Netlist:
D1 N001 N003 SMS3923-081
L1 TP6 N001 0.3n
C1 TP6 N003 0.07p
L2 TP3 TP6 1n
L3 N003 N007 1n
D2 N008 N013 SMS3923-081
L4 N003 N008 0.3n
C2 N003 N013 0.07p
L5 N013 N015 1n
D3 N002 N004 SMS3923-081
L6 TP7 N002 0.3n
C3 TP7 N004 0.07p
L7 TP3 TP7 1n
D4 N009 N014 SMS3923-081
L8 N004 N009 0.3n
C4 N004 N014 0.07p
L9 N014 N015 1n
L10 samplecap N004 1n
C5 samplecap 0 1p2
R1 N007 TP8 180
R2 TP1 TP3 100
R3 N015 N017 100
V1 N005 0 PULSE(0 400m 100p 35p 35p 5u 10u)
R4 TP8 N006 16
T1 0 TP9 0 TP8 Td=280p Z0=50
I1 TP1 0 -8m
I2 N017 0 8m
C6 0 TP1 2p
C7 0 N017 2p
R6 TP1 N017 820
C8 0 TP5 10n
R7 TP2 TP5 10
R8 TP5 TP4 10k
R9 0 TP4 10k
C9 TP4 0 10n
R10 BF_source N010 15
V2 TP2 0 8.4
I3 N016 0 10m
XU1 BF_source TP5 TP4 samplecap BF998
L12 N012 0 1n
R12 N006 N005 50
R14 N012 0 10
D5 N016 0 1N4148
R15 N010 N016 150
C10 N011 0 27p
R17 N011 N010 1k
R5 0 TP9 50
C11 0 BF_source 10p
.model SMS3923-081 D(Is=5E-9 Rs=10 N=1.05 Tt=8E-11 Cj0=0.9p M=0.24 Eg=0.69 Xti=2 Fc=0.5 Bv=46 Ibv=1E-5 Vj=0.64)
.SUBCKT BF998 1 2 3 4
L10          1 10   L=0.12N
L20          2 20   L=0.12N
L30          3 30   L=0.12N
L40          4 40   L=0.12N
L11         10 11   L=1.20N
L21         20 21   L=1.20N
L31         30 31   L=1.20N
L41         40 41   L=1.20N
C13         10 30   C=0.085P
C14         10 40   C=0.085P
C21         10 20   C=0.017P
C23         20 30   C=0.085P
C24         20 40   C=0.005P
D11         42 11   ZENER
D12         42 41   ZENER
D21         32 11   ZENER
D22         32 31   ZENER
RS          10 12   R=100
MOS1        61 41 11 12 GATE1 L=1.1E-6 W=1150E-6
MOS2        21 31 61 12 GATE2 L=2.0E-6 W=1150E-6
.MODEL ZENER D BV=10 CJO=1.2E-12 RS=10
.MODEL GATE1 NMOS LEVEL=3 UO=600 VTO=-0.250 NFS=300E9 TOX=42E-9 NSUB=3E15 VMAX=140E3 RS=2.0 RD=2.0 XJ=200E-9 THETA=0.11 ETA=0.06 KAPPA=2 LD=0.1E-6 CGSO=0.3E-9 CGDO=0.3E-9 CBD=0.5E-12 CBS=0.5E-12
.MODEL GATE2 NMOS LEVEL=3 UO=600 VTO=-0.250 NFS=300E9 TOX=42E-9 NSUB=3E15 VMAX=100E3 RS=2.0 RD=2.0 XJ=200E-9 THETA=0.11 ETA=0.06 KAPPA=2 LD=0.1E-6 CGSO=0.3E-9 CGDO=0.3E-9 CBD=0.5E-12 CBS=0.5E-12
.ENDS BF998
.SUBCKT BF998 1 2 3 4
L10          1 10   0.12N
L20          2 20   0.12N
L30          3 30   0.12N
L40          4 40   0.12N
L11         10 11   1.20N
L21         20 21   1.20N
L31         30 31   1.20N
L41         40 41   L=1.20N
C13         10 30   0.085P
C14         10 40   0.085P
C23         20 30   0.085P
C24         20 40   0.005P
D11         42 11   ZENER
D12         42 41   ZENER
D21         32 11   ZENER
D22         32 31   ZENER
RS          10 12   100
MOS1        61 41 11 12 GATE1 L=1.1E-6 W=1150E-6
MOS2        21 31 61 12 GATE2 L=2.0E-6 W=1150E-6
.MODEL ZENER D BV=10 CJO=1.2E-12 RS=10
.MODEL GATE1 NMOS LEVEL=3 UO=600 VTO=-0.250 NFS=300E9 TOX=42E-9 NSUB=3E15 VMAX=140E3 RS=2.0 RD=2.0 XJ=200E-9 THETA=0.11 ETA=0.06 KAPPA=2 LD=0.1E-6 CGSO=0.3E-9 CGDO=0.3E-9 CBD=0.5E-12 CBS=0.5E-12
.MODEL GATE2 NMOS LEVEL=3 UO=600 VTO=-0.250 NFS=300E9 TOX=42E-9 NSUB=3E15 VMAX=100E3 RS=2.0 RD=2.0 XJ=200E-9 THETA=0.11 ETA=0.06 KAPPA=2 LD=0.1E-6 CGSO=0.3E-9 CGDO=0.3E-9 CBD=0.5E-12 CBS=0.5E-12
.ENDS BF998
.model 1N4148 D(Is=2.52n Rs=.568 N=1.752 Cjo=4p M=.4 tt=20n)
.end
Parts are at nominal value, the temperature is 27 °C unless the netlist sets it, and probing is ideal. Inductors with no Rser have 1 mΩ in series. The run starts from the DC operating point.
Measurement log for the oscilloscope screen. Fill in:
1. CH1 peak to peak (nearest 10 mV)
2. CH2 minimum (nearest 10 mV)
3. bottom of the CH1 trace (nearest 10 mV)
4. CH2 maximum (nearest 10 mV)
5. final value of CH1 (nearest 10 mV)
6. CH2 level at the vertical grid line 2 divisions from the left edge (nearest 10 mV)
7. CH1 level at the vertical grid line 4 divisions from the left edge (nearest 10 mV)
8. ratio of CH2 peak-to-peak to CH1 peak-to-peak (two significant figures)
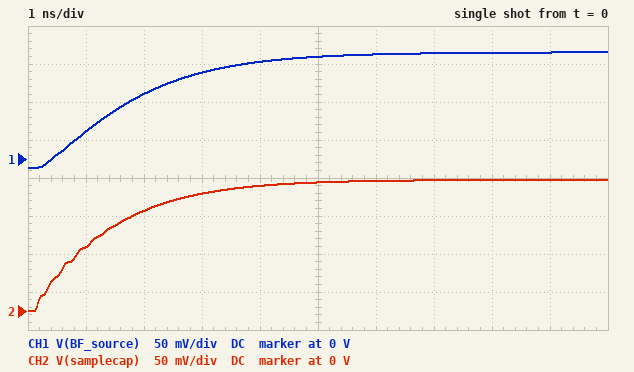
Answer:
150 mV
0 V
-10 mV
170 mV
140 mV
130 mV
130 mV
1.1
